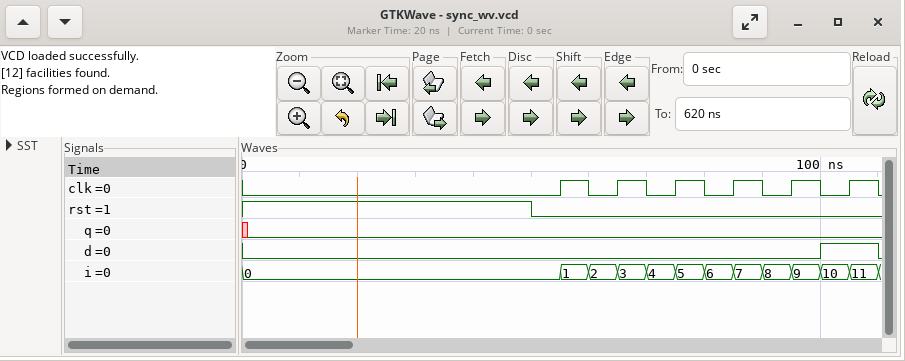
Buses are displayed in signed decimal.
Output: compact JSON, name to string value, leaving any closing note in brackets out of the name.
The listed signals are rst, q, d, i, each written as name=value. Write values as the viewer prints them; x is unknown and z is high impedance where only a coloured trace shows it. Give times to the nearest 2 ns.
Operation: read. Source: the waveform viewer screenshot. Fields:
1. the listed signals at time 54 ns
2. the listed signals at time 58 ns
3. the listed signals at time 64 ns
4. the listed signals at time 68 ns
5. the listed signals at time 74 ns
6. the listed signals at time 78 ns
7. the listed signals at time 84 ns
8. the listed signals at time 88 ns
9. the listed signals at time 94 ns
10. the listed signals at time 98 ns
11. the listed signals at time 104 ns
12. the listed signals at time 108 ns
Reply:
{"the listed signals at time 54 ns": "rst=0, q=0, d=0, i=0", "the listed signals at time 58 ns": "rst=0, q=0, d=0, i=1", "the listed signals at time 64 ns": "rst=0, q=0, d=0, i=2", "the listed signals at time 68 ns": "rst=0, q=0, d=0, i=3", "the listed signals at time 74 ns": "rst=0, q=0, d=0, i=4", "the listed signals at time 78 ns": "rst=0, q=0, d=0, i=5", "the listed signals at time 84 ns": "rst=0, q=0, d=0, i=6", "the listed signals at time 88 ns": "rst=0, q=0, d=0, i=7", "the listed signals at time 94 ns": "rst=0, q=0, d=0, i=8", "the listed signals at time 98 ns": "rst=0, q=0, d=0, i=9", "the listed signals at time 104 ns": "rst=0, q=0, d=1, i=10", "the listed signals at time 108 ns": "rst=0, q=0, d=1, i=11"}
